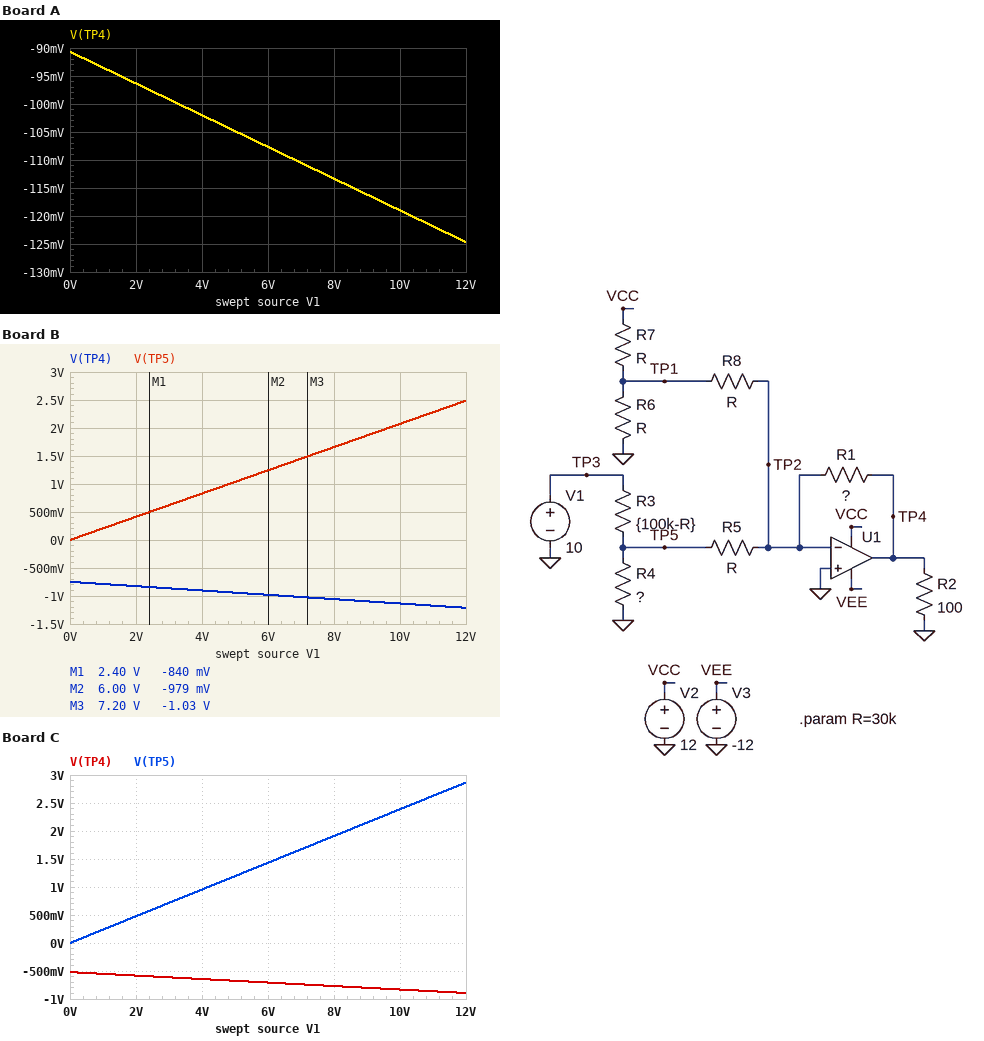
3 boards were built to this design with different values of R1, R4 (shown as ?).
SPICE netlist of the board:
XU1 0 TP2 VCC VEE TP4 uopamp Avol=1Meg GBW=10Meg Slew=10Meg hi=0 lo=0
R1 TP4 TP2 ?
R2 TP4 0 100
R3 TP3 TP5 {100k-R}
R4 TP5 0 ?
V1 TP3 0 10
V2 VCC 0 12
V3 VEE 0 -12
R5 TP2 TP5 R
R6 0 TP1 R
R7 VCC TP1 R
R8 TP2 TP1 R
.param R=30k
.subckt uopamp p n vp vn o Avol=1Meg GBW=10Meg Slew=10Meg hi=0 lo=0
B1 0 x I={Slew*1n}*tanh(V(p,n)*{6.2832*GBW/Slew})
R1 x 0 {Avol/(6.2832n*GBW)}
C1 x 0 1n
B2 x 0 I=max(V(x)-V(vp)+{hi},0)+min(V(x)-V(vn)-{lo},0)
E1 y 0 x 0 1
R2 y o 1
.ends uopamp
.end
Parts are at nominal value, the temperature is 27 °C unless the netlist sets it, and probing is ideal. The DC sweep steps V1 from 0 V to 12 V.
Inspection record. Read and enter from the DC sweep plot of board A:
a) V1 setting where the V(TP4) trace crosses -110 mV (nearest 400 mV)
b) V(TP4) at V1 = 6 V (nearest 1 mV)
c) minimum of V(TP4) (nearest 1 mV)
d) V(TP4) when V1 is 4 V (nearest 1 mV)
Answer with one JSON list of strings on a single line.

["6.8 V", "-108 mV", "-125 mV", "-102 mV"]
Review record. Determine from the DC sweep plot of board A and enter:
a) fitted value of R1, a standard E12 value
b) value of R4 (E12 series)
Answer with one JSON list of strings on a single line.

["680 Ω", "15 kΩ"]
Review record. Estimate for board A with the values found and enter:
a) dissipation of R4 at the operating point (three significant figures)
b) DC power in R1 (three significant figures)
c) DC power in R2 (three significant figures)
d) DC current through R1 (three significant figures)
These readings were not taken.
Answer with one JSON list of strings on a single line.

["104 µW", "20.8 µW", "142 µW", "175 µA"]
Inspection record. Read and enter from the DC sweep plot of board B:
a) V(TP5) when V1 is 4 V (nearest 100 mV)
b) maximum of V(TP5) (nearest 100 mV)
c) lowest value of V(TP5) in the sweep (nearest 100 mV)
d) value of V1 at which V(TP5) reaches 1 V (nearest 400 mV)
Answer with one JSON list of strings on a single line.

["800 mV", "2.5 V", "0 V", "4.8 V"]
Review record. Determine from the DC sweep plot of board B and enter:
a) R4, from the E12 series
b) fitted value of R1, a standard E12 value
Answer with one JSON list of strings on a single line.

["47 kΩ", "5.6 kΩ"]
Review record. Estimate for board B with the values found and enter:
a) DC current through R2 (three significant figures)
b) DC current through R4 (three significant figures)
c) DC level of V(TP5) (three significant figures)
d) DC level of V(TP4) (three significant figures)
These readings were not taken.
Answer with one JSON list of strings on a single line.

["11.3 mA", "44.1 µA", "2.07 V", "-1.13 V"]
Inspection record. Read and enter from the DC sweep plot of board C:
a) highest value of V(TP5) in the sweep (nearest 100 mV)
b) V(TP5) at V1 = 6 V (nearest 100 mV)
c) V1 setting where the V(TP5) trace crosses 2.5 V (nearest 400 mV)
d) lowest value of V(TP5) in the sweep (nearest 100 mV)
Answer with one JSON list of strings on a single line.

["2.9 V", "1.4 V", "10.4 V", "0 V"]
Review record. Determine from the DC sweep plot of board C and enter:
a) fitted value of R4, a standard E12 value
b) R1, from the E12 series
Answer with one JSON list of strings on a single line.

["82 kΩ", "3.9 kΩ"]
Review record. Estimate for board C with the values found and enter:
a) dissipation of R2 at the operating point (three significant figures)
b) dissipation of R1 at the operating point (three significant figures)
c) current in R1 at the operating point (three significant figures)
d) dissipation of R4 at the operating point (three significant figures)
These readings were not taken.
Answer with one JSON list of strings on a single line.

["6.90 mW", "177 µW", "213 µA", "69.6 µW"]
